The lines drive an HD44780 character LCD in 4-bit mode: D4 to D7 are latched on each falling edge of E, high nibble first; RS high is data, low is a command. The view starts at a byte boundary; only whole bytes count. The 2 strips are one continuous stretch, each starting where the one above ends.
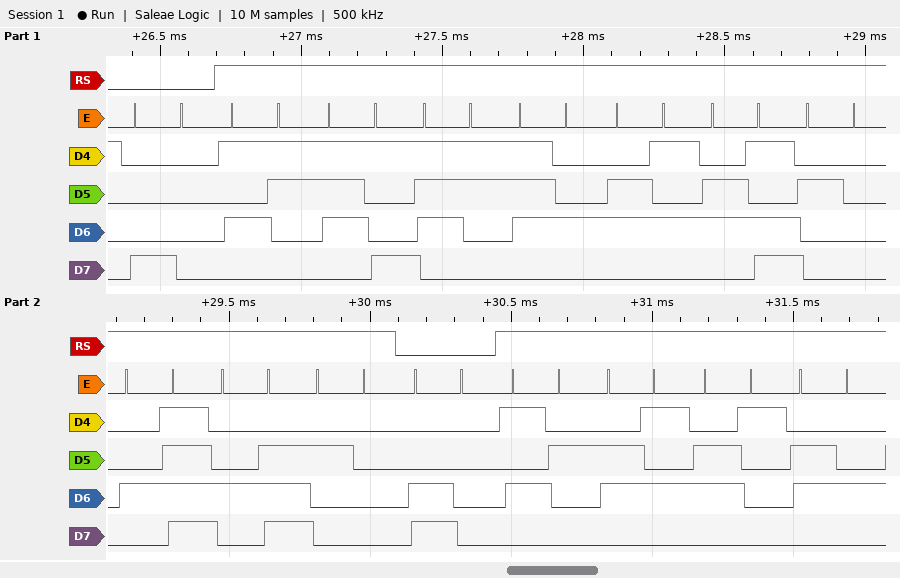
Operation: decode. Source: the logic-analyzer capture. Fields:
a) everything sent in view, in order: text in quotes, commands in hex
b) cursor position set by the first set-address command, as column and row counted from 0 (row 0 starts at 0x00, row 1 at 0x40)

0x80 "System ON " 0xC0 "Read"
column 0, row 0
